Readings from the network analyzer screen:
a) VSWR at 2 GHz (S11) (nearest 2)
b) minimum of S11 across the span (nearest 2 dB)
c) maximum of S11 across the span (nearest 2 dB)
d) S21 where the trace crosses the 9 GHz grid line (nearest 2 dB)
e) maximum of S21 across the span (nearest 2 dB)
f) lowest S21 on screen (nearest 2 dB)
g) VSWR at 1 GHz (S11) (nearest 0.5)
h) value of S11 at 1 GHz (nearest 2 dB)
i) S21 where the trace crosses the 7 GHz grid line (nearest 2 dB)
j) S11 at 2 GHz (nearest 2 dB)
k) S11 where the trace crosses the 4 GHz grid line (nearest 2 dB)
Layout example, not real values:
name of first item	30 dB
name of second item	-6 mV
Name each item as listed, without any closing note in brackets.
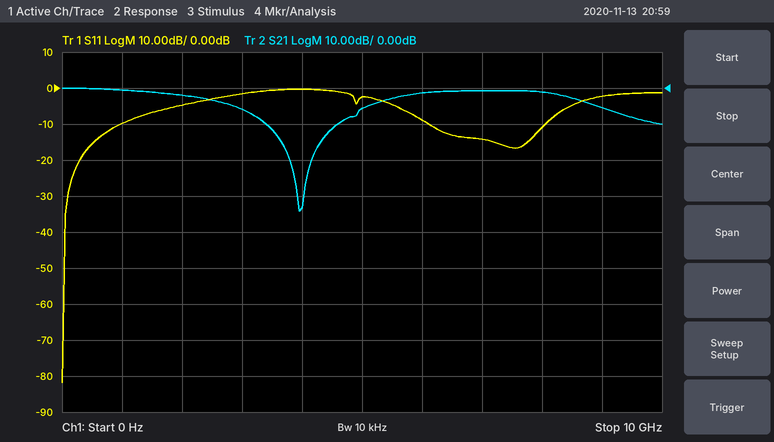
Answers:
VSWR at 2 GHz (S11)	4
minimum of S11 across the span	-82 dB
maximum of S11 across the span	0 dB
S21 where the trace crosses the 9 GHz grid line	-6 dB
maximum of S21 across the span	0 dB
lowest S21 on screen	-34 dB
VSWR at 1 GHz (S11)	2.0
value of S11 at 1 GHz	-10 dB
S21 where the trace crosses the 7 GHz grid line	0 dB
S11 at 2 GHz	-4 dB
S11 where the trace crosses the 4 GHz grid line	0 dB
